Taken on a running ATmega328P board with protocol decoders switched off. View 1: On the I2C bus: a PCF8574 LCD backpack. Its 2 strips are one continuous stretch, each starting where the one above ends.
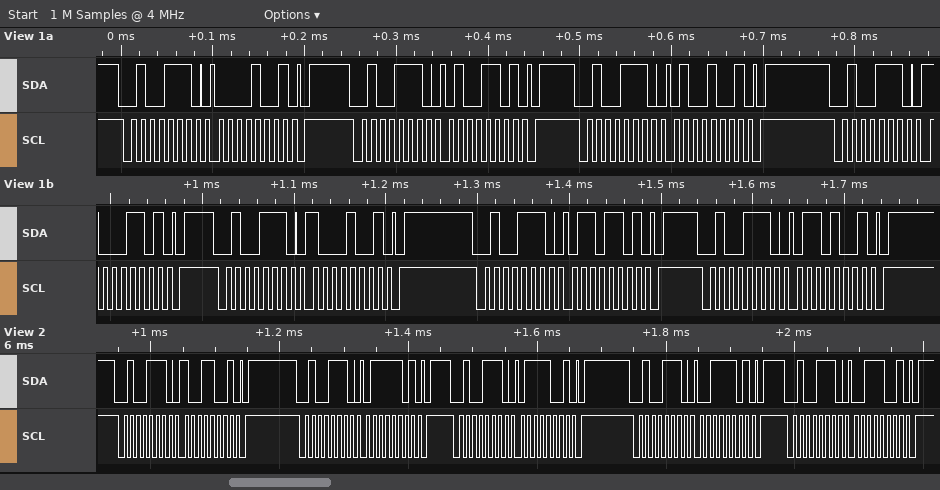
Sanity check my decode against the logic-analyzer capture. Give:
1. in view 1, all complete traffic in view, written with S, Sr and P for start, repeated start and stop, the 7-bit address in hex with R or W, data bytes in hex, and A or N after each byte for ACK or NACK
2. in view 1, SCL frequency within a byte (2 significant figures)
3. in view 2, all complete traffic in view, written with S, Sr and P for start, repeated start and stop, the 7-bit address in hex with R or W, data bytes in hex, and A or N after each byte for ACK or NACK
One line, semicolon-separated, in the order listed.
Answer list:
S 27W A 09 A P S 27W A 4D A P S 27W A 49 A P S 27W A 8D A P S 27W A 89 A P S 27W A 6D A P S 27W A 69 A P; 100 kHz; S 27W A 99 A P S 27W A 7D A P S 27W A 79 A P S 27W A 3D A P S 27W A 39 A P
